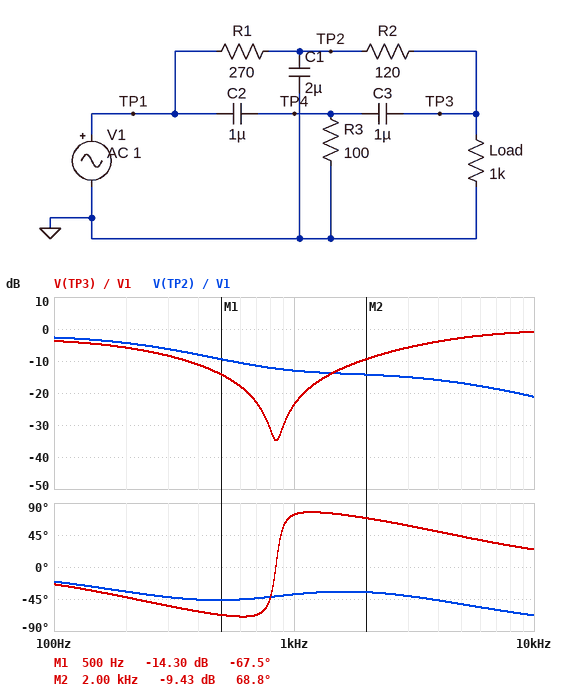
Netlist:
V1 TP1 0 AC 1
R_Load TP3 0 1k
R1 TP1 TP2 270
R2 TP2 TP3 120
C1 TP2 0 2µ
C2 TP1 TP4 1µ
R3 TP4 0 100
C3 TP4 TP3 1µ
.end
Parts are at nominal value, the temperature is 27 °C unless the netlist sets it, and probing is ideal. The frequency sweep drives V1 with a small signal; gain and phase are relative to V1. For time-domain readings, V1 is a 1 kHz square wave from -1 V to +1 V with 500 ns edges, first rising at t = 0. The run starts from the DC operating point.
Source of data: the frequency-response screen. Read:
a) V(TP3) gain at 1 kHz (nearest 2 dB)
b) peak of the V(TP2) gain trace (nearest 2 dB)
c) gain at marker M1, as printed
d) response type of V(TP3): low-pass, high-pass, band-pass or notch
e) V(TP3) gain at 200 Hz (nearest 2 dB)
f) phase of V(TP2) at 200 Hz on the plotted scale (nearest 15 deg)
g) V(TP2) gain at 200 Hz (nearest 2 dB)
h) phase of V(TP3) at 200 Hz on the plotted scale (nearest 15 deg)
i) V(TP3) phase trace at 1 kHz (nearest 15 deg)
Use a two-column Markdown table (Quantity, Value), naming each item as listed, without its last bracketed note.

| Quantity | Value |
|---|---|
| V(TP3) gain at 1 kHz | -24 dB |
| peak of the V(TP2) gain trace | -2 dB |
| gain at marker M1, as printed | -14.30 dB |
| response type of V(TP3): low-pass, high-pass, band-pass or notch | notch |
| V(TP3) gain at 200 Hz | -6 dB |
| phase of V(TP2) at 200 Hz on the plotted scale | -30 deg |
| V(TP2) gain at 200 Hz | -4 dB |
| phase of V(TP3) at 200 Hz on the plotted scale | -45 deg |
| V(TP3) phase trace at 1 kHz | 75 deg |
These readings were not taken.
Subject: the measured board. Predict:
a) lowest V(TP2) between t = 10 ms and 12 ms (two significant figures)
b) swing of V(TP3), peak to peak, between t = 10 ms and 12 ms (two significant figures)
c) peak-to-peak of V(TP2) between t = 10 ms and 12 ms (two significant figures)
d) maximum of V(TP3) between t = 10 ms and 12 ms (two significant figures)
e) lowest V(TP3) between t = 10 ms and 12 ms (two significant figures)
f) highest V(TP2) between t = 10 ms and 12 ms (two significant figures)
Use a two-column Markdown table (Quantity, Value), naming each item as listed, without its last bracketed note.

| Quantity | Value |
|---|---|
| lowest V(TP2) between t = 10 ms and 12 ms | -340 mV |
| swing of V(TP3), peak to peak, between t = 10 ms and 12 ms | 3.6 V |
| peak-to-peak of V(TP2) between t = 10 ms and 12 ms | 690 mV |
| maximum of V(TP3) between t = 10 ms and 12 ms | 1.8 V |
| lowest V(TP3) between t = 10 ms and 12 ms | -1.8 V |
| highest V(TP2) between t = 10 ms and 12 ms | 340 mV |
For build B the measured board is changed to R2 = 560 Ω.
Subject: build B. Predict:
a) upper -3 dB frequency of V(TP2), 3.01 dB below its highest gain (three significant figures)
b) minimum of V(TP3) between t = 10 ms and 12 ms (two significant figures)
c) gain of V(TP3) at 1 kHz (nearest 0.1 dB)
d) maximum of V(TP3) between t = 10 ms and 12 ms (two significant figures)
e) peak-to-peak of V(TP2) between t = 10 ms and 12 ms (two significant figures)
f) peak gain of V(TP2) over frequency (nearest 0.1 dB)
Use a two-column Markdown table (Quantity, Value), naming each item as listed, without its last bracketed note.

| Quantity | Value |
|---|---|
| upper -3 dB frequency of V(TP2), 3.01 dB below its highest gain | 265 Hz |
| minimum of V(TP3) between t = 10 ms and 12 ms | -2.0 V |
| gain of V(TP3) at 1 kHz | -9.9 dB |
| maximum of V(TP3) between t = 10 ms and 12 ms | 2.0 V |
| peak-to-peak of V(TP2) between t = 10 ms and 12 ms | 830 mV |
| peak gain of V(TP2) over frequency | -1.4 dB |
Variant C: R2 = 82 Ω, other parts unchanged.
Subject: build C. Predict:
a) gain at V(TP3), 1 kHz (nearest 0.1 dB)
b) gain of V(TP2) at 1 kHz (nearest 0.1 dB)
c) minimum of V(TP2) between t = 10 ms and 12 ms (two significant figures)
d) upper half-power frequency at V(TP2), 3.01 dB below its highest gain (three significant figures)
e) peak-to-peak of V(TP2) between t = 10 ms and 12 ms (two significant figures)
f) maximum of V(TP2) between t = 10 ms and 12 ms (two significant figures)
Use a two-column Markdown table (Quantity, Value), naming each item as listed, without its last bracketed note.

| Quantity | Value |
|---|---|
| gain at V(TP3), 1 kHz | -26.7 dB |
| gain of V(TP2) at 1 kHz | -13.6 dB |
| minimum of V(TP2) between t = 10 ms and 12 ms | -330 mV |
| upper half-power frequency at V(TP2), 3.01 dB below its highest gain | 223 Hz |
| peak-to-peak of V(TP2) between t = 10 ms and 12 ms | 660 mV |
| maximum of V(TP2) between t = 10 ms and 12 ms | 330 mV |
